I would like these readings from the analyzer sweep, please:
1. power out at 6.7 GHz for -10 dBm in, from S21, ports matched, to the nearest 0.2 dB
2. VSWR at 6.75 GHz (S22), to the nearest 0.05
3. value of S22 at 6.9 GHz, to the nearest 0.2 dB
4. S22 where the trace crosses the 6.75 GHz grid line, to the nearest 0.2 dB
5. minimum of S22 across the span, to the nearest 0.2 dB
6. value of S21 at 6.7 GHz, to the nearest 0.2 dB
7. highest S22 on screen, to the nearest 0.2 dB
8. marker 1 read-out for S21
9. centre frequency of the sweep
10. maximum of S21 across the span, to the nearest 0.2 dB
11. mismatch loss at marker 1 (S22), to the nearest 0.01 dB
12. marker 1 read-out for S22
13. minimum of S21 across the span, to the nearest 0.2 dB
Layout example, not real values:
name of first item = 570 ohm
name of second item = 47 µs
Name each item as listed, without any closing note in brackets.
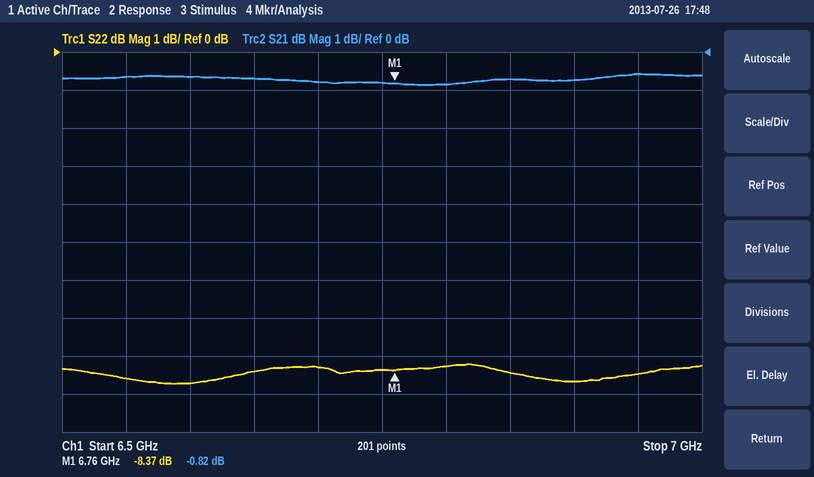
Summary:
power out at 6.7 GHz for -10 dBm in, from S21, ports matched, to the nearest 0.2 dB = -10.8 dBm
VSWR at 6.75 GHz (S22), to the nearest 0.05 = 2.25
value of S22 at 6.9 GHz, to the nearest 0.2 dB = -8.6 dB
S22 where the trace crosses the 6.75 GHz grid line, to the nearest 0.2 dB = -8.4 dB
minimum of S22 across the span, to the nearest 0.2 dB = -8.8 dB
value of S21 at 6.7 GHz, to the nearest 0.2 dB = -0.8 dB
highest S22 on screen, to the nearest 0.2 dB = -8.2 dB
marker 1 read-out for S21 = -0.82 dB
centre frequency of the sweep = 6.75 GHz
maximum of S21 across the span, to the nearest 0.2 dB = -0.6 dB
mismatch loss at marker 1 (S22), to the nearest 0.01 dB = 0.68 dB
marker 1 read-out for S22 = -8.37 dB
minimum of S21 across the span, to the nearest 0.2 dB = -0.8 dB
